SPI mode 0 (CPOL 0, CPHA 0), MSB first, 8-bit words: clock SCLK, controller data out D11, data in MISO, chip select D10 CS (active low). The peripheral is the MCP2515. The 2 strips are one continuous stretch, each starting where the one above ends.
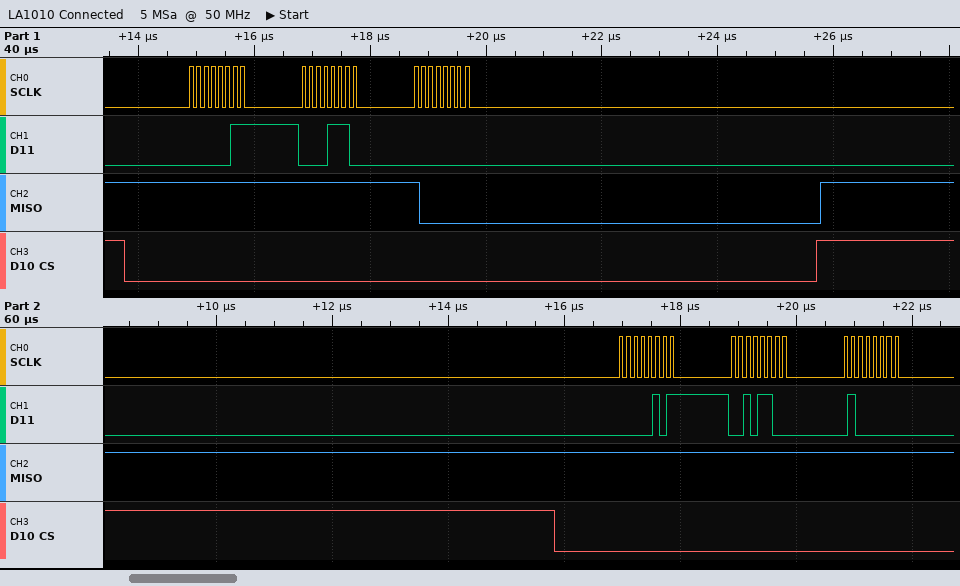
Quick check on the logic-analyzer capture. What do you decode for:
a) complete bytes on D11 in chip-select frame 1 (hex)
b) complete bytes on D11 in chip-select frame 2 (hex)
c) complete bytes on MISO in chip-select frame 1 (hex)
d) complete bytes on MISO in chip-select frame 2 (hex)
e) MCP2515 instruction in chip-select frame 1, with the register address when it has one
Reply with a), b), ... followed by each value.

a) 0x03 0x0E 0x00
b) 0x05 0x2C 0x40
c) 0xFF 0xFF 0x80
d) 0xFF 0xFF 0xFF
e) READ 0x0E
